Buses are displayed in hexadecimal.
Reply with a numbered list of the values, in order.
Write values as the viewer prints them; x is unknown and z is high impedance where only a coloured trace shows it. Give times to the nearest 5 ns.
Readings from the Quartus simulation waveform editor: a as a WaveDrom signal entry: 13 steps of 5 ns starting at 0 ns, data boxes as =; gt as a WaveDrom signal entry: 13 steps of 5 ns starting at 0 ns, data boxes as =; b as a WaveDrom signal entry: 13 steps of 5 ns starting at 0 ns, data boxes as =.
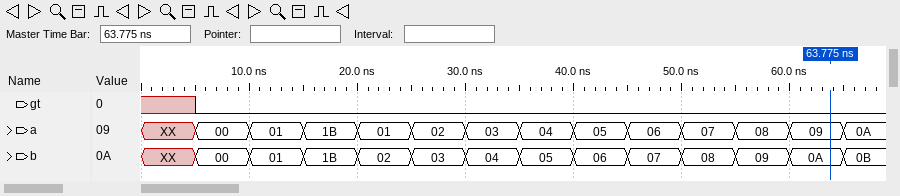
1. {name: 'a', wave: 'x============', data: '00 01 1B 01 02 03 04 05 06 07 08 09'}
2. {name: 'gt', wave: 'x0...........'}
3. {name: 'b', wave: 'x============', data: '00 01 1B 02 03 04 05 06 07 08 09 0A'}
